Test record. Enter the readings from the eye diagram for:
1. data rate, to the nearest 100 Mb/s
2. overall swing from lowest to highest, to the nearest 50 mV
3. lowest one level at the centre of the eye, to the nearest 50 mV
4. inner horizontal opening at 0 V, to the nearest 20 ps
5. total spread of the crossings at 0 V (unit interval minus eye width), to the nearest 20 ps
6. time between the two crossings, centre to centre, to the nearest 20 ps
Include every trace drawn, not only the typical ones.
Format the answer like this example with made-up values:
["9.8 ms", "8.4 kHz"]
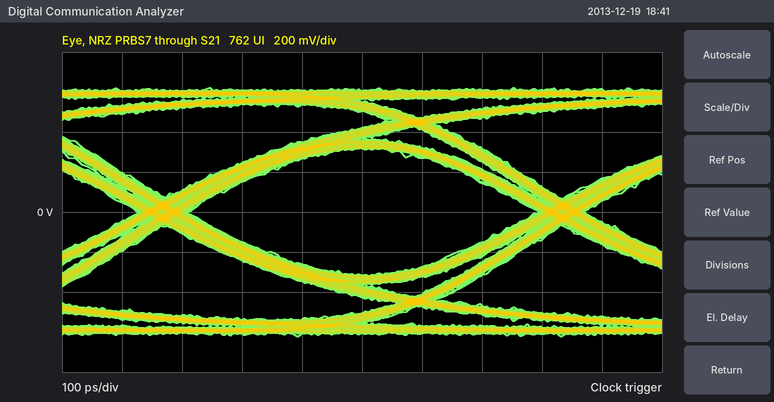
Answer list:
["1.5 Gb/s", "1.25 V", "300 mV", "580 ps", "80 ps", "660 ps"]
